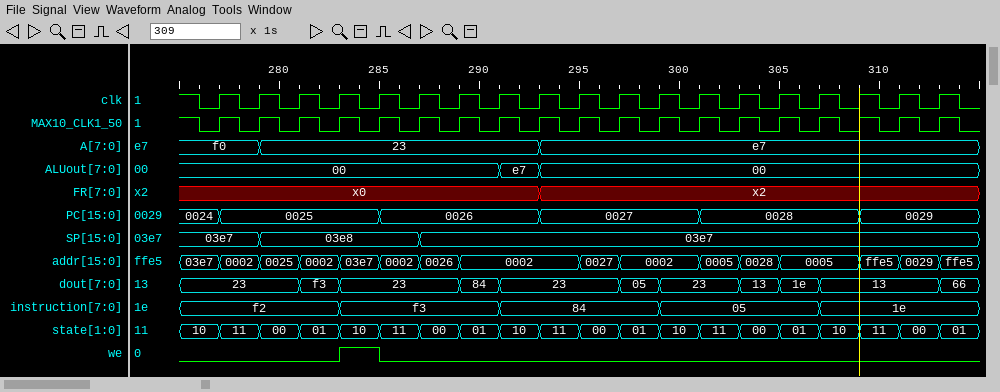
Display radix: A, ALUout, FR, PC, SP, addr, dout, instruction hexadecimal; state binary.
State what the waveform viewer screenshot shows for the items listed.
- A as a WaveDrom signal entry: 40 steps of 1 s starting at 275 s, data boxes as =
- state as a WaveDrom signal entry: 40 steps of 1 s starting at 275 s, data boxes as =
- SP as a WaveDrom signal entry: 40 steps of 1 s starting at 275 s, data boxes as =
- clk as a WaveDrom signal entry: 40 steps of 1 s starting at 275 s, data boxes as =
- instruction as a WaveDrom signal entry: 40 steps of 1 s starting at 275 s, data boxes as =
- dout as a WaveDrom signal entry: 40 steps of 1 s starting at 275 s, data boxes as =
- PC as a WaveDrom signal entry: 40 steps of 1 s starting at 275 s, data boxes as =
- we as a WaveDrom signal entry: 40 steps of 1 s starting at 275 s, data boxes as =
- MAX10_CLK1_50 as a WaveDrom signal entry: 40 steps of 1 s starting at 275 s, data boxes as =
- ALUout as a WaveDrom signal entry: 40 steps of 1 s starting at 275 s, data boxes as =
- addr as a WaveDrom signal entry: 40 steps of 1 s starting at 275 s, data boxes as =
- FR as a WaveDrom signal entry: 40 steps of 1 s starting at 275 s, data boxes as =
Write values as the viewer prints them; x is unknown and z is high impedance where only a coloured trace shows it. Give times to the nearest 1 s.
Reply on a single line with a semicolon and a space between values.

{name: 'A', wave: '=...=.............=.....................', data: 'f0 23 e7'}; {name: 'state', wave: '=.=.=.=.=.=.=.=.=.=.=.=.=.=.=.=.=.=.=.=.', data: '10 11 00 01 10 11 00 01 10 11 00 01 10 11 00 01 10 11 00 01'}; {name: 'SP', wave: '=...=.......=...........................', data: '03e7 03e8 03e7'}; {name: 'clk', wave: '1010101010101010101010101010101010101010'}; {name: 'instruction', wave: '=.......=.......=.......=.......=.......', data: 'f2 f3 84 05 1e'}; {name: 'dout', wave: '=.....=.=.....=.=.....=.=...=.=.=.....=.', data: '23 f3 23 84 23 05 23 13 1e 13 66'}; {name: 'PC', wave: '=.=.......=.......=.......=.......=.....', data: '0024 0025 0026 0027 0028 0029'}; {name: 'we', wave: '0.......1.0.............................'}; {name: 'MAX10_CLK1_50', wave: '1010101010101010101010101010101010101010'}; {name: 'ALUout', wave: '=...............=.=.....................', data: '00 e7 00'}; {name: 'addr', wave: '=.=.=.=.=.=.=.=.....=.=...=.=.=...=.=.=.', data: '03e7 0002 0025 0002 03e7 0002 0026 0002 0027 0002 0005 0028 0005 ffe5 0029 ffe5'}; {name: 'FR', wave: '=.................=.....................', data: 'x0 x2'}
